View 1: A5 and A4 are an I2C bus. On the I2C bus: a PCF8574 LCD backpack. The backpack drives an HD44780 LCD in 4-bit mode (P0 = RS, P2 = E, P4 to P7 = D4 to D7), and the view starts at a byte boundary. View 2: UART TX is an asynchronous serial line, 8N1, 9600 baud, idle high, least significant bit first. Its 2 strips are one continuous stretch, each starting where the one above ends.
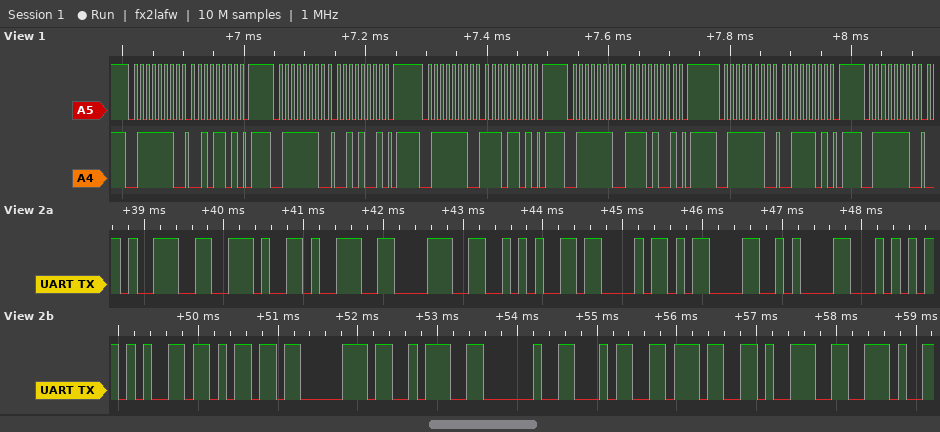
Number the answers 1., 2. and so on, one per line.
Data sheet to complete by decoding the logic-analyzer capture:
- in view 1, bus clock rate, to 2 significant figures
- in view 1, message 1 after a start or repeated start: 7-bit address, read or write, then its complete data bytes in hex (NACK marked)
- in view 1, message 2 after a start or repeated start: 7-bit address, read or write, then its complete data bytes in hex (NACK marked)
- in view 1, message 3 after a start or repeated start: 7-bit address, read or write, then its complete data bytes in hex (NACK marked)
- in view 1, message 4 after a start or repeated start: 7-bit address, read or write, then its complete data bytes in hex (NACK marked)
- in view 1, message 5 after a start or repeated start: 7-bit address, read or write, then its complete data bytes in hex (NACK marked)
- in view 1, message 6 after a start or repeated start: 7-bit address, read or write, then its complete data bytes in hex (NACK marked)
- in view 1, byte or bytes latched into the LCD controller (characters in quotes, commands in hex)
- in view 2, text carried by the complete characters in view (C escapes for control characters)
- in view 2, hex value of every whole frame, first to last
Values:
1. 100 kHz
2. 0x3F write: 2D
3. 0x3F write: 29
4. 0x3F write: ED
5. 0x3F write: E9
6. 0x3F write: 3D
7. 0x3F write
8. '.'
9. "9.98*C\r\nTemp: 479."
10. 39 2E 39 38 2A 43 0D 0A 54 65 6D 70 3A 20 34 37 39 2E
